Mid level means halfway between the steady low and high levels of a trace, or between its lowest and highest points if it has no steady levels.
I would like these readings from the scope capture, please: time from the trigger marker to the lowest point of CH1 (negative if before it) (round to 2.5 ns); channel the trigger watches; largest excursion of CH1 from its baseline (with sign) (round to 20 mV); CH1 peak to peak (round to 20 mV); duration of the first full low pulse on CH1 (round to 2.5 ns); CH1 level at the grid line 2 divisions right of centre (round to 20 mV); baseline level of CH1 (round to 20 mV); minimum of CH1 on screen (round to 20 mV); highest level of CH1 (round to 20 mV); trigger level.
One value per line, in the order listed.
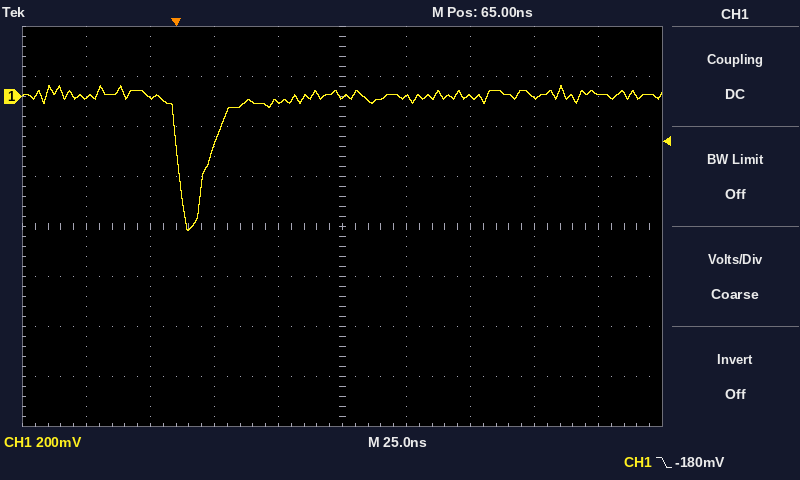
+5.0 ns
CH1
-540 mV
580 mV
12.5 ns
0 mV
0 mV
-540 mV
40 mV
-180 mV
